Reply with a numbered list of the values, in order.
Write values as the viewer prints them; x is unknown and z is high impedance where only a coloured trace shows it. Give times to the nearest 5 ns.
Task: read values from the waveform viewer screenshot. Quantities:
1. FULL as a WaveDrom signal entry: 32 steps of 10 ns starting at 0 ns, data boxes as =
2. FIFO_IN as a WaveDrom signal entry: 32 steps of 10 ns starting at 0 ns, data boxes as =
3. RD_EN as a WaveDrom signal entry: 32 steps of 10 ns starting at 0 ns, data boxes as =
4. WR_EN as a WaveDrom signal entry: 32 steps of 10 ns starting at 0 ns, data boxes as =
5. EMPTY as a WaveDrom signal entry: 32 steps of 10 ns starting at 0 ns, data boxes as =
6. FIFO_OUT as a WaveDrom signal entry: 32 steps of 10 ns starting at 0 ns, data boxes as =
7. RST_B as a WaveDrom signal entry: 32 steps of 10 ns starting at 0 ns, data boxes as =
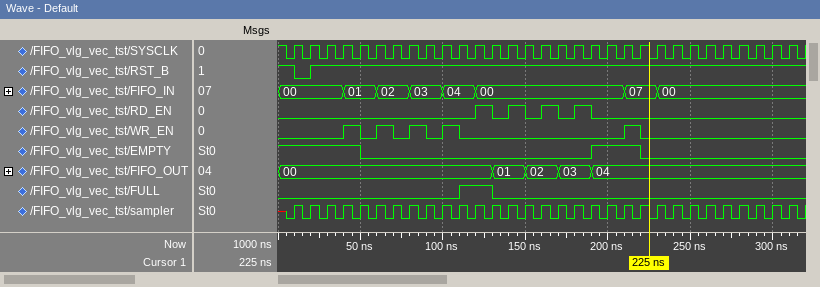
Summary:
1. {name: 'FULL', wave: '0..........1.0..................'}
2. {name: 'FIFO_IN', wave: '=...=.=.=.=.=........=.=........', data: '00 01 02 03 04 00 07 00'}
3. {name: 'RD_EN', wave: '0...........10101010............'}
4. {name: 'WR_EN', wave: '0...10101010.........10.........'}
5. {name: 'EMPTY', wave: '1....0.............1..0.........'}
6. {name: 'FIFO_OUT', wave: '=............=.=.=.=............', data: '00 01 02 03 04'}
7. {name: 'RST_B', wave: '101.............................'}
